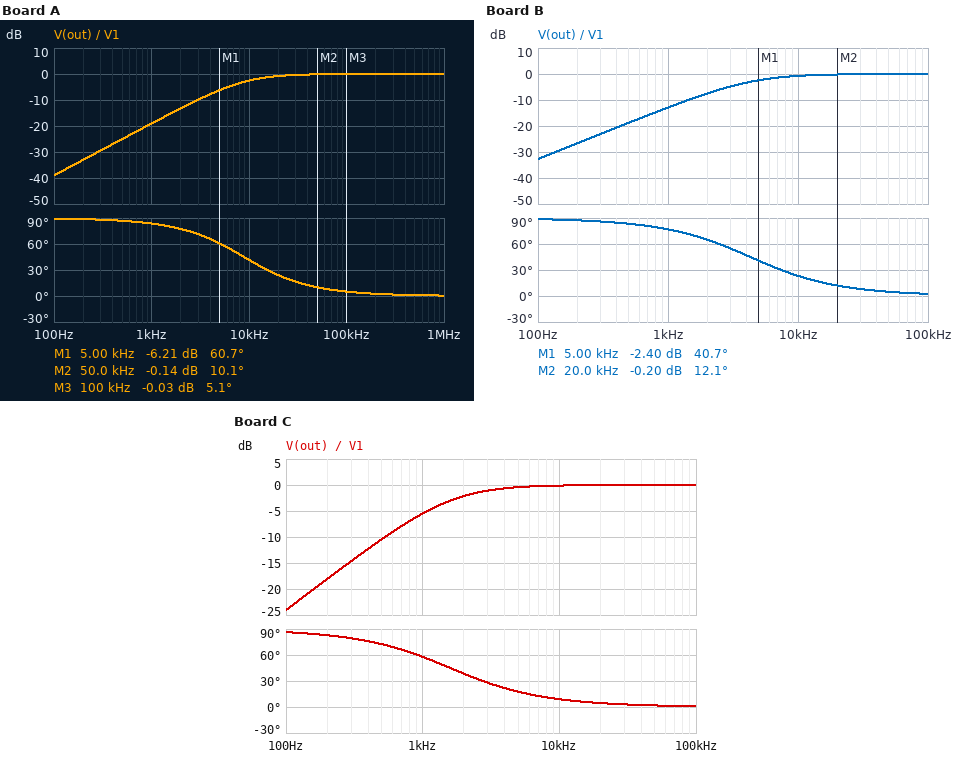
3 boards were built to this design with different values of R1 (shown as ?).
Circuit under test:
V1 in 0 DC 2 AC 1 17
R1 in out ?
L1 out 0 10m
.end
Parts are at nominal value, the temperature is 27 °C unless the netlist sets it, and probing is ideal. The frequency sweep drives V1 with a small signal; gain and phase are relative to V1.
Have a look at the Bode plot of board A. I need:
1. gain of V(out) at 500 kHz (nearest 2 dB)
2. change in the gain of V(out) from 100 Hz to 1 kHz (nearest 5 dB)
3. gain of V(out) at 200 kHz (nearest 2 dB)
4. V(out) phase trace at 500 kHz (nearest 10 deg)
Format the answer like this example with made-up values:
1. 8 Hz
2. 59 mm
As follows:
1. 0 dB
2. 20 dB
3. 0 dB
4. 0 deg
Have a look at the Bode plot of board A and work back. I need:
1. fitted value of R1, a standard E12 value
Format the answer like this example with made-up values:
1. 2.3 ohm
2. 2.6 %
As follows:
1. 560 Ω
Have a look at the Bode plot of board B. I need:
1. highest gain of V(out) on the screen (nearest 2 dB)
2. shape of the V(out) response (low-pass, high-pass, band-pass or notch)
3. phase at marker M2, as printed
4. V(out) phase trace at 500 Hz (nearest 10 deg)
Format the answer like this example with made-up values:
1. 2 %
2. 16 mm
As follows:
1. 0 dB
2. high-pass
3. 12.1 deg
4. 80 deg
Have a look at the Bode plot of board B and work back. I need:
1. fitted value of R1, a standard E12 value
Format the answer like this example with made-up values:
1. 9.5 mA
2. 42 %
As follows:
1. 270 Ω
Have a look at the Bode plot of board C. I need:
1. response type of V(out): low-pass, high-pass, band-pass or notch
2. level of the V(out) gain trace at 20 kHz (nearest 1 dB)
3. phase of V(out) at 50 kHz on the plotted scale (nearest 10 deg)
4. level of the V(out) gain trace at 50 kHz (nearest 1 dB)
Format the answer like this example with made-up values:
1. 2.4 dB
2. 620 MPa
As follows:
1. high-pass
2. 0 dB
3. 0 deg
4. 0 dB
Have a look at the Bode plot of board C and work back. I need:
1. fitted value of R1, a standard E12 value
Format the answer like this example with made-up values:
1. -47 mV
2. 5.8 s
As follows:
1. 100 Ω
